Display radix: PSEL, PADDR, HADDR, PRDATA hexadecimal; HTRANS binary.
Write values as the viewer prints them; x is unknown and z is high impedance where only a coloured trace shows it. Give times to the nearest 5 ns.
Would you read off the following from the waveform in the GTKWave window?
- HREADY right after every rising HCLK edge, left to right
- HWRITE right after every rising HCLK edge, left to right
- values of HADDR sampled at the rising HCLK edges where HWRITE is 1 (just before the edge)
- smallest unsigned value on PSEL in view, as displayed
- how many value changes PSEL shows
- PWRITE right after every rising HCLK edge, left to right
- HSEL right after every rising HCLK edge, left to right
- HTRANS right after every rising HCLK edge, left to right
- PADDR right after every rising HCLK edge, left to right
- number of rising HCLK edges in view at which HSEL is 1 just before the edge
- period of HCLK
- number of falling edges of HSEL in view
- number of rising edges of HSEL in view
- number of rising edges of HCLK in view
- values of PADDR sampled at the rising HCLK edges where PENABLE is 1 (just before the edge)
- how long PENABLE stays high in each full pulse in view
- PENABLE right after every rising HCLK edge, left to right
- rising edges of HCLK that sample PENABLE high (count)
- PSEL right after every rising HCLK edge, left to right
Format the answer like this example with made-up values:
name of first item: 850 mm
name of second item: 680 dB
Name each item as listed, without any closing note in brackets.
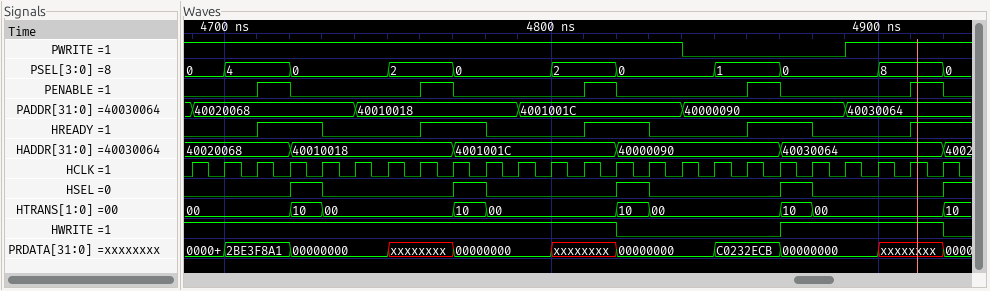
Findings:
HREADY right after every rising HCLK edge, left to right: 0 0 1 1 0 0 0 1 1 0 0 0 1 1 0 0 0 1 1 0 0 0 1 1
HWRITE right after every rising HCLK edge, left to right: 1 1 1 1 1 1 1 1 1 1 1 1 1 0 0 0 0 0 1 1 1 1 1 0
values of HADDR sampled at the rising HCLK edges where HWRITE is 1: 40020068, 40020068, 40020068, 40020068, 40010018, 40010018, 40010018, 40010018, 40010018, 4001001C, 4001001C, 4001001C, 4001001C, 4001001C, 40030064, 40030064, 40030064, 40030064, 40030064
smallest unsigned value on PSEL in view, as displayed: 0
how many value changes PSEL shows: 10
PWRITE right after every rising HCLK edge, left to right: 1 1 1 1 1 1 1 1 1 1 1 1 1 1 1 0 0 0 0 0 1 1 1 1
HSEL right after every rising HCLK edge, left to right: 0 0 0 1 0 0 0 0 1 0 0 0 0 1 0 0 0 0 1 0 0 0 0 1
HTRANS right after every rising HCLK edge, left to right: 00, 00, 00, 10, 00, 00, 00, 00, 10, 00, 00, 00, 00, 10, 00, 00, 00, 00, 10, 00, 00, 00, 00, 10
PADDR right after every rising HCLK edge, left to right: 40020068, 40020068, 40020068, 40020068, 40020068, 40010018, 40010018, 40010018, 40010018, 40010018, 4001001C, 4001001C, 4001001C, 4001001C, 4001001C, 40000090, 40000090, 40000090, 40000090, 40000090, 40030064, 40030064, 40030064, 40030064
number of rising HCLK edges in view at which HSEL is 1 just before the edge: 4
period of HCLK: 10 ns
number of falling edges of HSEL in view: 4
number of rising edges of HSEL in view: 5
number of rising edges of HCLK in view: 24
values of PADDR sampled at the rising HCLK edges where PENABLE is 1: 40020068, 40010018, 4001001C, 40000090, 40030064
how long PENABLE stays high in each full pulse in view: 10 ns, 10 ns, 10 ns, 10 ns, 10 ns
PENABLE right after every rising HCLK edge, left to right: 0 0 1 0 0 0 0 1 0 0 0 0 1 0 0 0 0 1 0 0 0 0 1 0
rising edges of HCLK that sample PENABLE high: 5
PSEL right after every rising HCLK edge, left to right: 0, 4, 4, 0, 0, 0, 2, 2, 0, 0, 0, 2, 2, 0, 0, 0, 1, 1, 0, 0, 0, 8, 8, 0
